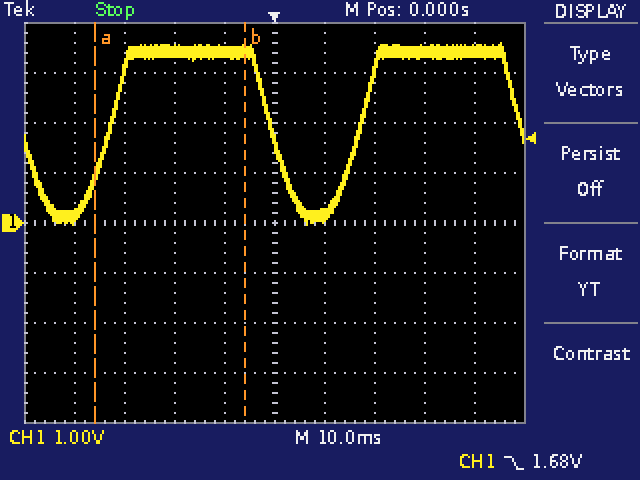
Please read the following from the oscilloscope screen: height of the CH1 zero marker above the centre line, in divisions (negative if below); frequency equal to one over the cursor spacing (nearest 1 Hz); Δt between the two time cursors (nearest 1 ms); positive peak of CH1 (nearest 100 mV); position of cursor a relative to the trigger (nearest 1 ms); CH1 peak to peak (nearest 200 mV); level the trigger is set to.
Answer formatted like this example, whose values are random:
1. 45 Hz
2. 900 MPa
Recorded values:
1. 0.0 div
2. 33 Hz
3. 30 ms
4. 3.6 V
5. -36 ms
6. 3.6 V
7. 1.68 V
